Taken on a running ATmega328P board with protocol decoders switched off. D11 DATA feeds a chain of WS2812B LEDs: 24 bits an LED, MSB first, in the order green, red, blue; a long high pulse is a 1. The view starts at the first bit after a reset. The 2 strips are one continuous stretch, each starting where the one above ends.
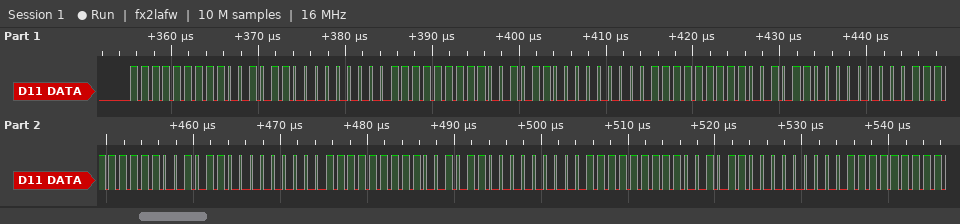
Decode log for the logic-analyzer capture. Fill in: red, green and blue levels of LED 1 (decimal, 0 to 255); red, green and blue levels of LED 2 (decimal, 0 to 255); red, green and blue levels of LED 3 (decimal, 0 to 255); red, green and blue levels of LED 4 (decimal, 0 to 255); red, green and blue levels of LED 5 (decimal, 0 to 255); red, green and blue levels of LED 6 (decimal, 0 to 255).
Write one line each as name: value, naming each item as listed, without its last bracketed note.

red, green and blue levels of LED 1: 150, 255, 0
red, green and blue levels of LED 2: 150, 255, 0
red, green and blue levels of LED 3: 150, 255, 0
red, green and blue levels of LED 4: 150, 255, 0
red, green and blue levels of LED 5: 150, 255, 0
red, green and blue levels of LED 6: 150, 255, 0
